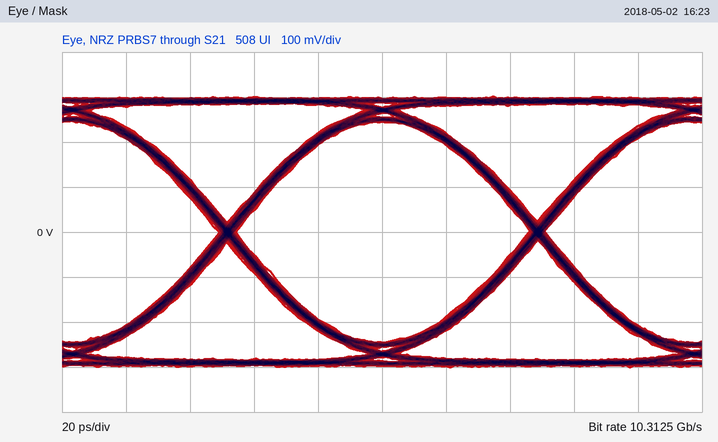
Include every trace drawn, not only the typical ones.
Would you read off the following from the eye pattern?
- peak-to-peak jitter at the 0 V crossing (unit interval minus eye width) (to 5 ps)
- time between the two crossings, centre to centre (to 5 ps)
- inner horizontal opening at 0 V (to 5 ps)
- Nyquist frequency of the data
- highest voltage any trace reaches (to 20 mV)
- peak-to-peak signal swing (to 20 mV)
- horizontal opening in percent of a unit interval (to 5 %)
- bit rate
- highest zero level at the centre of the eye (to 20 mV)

5 ps
95 ps
90 ps
5.15625 GHz
300 mV
600 mV
95 %
10.3125 Gb/s
-240 mV
